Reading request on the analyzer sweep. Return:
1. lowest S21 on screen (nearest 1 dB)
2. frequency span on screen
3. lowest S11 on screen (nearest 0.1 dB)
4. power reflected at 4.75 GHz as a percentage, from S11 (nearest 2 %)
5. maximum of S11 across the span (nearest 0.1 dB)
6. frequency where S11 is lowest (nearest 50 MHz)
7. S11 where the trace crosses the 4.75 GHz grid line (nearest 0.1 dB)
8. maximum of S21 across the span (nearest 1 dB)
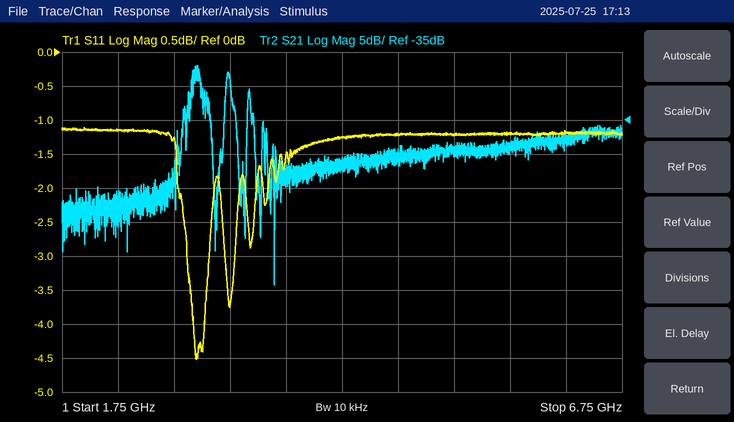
-59 dB
5 GHz
-4.5 dB
76 %
-1.1 dB
2.95 GHz
-1.2 dB
-27 dB
